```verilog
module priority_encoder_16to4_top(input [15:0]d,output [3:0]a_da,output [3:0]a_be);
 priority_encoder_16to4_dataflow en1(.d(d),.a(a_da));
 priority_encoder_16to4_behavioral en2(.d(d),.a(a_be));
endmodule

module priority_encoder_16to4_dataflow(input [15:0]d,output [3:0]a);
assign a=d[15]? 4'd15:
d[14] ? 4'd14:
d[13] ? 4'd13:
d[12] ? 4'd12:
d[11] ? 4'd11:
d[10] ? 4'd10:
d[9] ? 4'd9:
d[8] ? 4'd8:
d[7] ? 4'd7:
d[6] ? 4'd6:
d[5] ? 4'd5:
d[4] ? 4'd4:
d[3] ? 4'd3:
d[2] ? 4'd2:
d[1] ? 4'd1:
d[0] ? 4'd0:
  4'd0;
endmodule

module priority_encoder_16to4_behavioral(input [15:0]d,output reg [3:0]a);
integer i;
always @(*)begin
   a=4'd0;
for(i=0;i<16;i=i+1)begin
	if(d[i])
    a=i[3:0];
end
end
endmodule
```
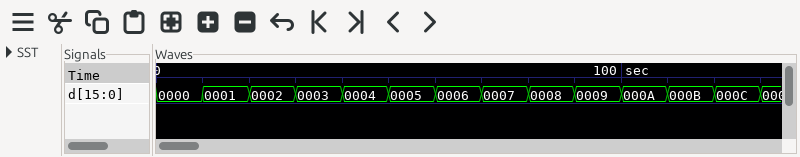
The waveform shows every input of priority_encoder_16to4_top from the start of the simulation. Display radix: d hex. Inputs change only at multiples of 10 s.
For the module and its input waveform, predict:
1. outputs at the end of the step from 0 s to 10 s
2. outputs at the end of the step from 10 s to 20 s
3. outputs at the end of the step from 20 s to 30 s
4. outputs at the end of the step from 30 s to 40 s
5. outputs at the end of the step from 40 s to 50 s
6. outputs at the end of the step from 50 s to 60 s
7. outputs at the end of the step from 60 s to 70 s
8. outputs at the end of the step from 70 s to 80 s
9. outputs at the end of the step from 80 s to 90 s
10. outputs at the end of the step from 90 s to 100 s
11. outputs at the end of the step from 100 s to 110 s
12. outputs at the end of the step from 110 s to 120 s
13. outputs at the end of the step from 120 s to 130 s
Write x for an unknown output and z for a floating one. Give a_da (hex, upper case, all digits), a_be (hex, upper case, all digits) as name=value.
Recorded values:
a_da=0, a_be=0
a_da=0, a_be=0
a_da=1, a_be=1
a_da=1, a_be=1
a_da=2, a_be=2
a_da=2, a_be=2
a_da=2, a_be=2
a_da=2, a_be=2
a_da=3, a_be=3
a_da=3, a_be=3
a_da=3, a_be=3
a_da=3, a_be=3
a_da=3, a_be=3
